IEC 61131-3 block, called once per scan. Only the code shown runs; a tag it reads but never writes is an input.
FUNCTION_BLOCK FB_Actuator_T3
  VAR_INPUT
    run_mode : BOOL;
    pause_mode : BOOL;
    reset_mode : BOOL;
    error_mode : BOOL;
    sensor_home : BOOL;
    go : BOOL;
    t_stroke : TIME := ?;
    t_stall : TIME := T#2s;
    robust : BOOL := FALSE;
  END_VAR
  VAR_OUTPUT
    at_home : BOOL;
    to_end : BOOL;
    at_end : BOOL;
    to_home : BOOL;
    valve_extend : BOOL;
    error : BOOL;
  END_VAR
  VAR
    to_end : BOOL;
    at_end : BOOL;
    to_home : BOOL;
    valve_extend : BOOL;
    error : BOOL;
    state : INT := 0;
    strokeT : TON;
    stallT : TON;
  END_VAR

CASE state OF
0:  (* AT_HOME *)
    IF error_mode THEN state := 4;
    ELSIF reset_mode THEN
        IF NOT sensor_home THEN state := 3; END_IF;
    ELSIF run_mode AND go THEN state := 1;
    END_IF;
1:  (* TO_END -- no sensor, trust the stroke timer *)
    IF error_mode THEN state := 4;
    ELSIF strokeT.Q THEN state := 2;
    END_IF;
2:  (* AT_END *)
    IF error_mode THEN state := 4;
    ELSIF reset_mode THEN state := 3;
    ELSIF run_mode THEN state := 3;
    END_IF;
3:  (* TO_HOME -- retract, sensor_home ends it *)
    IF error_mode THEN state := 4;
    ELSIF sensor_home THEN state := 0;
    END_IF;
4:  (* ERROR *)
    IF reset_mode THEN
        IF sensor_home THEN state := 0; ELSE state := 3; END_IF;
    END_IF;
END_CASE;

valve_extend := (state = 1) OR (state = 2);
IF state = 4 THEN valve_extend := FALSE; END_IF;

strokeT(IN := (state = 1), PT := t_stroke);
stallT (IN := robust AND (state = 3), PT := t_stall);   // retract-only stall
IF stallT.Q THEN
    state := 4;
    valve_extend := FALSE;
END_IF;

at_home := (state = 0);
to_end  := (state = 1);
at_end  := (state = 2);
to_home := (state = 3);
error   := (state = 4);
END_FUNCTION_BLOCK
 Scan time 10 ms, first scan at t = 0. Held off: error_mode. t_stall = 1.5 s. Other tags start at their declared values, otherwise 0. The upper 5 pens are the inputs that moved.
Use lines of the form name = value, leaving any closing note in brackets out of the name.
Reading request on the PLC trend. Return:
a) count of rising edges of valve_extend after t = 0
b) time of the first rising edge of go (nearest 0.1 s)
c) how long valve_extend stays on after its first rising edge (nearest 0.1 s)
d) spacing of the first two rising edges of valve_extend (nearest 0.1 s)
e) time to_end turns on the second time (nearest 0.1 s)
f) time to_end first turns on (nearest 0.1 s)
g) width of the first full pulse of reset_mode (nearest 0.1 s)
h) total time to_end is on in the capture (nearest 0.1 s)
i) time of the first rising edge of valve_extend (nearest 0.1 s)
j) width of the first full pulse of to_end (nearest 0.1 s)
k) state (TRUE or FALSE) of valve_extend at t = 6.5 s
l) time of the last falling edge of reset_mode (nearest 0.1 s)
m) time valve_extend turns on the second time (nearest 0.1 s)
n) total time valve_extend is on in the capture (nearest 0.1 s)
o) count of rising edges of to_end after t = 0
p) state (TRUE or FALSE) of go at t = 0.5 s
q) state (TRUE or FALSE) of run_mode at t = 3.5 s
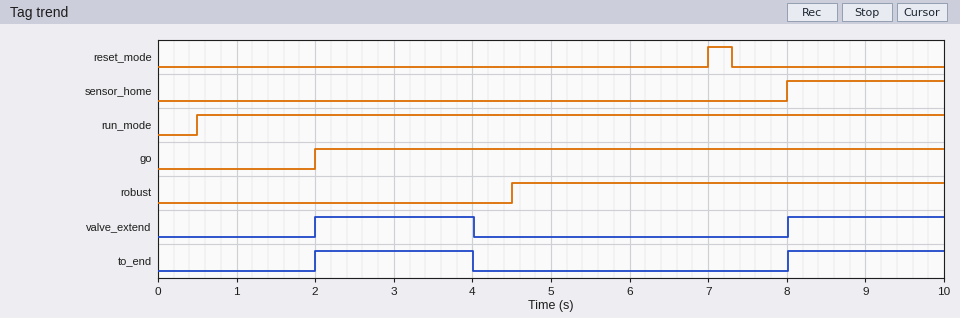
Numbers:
count of rising edges of valve_extend after t = 0 = 2
time of the first rising edge of go = 2.0 s
how long valve_extend stays on after its first rising edge = 2.0 s
spacing of the first two rising edges of valve_extend = 6.0 s
time to_end turns on the second time = 8.0 s
time to_end first turns on = 2.0 s
width of the first full pulse of reset_mode = 0.3 s
total time to_end is on in the capture = 4.0 s
time of the first rising edge of valve_extend = 2.0 s
width of the first full pulse of to_end = 2.0 s
state (TRUE or FALSE) of valve_extend at t = 6.5 s = FALSE
time of the last falling edge of reset_mode = 7.3 s
time valve_extend turns on the second time = 8.0 s
total time valve_extend is on in the capture = 4.0 s
count of rising edges of to_end after t = 0 = 2
state (TRUE or FALSE) of go at t = 0.5 s = FALSE
state (TRUE or FALSE) of run_mode at t = 3.5 s = TRUE
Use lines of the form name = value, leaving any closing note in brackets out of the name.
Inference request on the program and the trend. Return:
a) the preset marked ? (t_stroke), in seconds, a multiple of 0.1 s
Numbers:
the preset marked ? (t_stroke), in seconds, a multiple of 0.1 s = 2.0 s
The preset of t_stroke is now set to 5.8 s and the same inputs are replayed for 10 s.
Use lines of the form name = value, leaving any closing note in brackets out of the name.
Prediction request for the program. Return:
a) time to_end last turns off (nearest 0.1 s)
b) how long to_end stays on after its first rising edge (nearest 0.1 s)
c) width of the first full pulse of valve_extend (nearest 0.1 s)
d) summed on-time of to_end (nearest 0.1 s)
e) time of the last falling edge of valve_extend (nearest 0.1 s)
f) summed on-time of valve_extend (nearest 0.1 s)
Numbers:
time to_end last turns off = 7.8 s
how long to_end stays on after its first rising edge = 5.8 s
width of the first full pulse of valve_extend = 5.8 s
summed on-time of to_end = 7.8 s
time of the last falling edge of valve_extend = 7.8 s
summed on-time of valve_extend = 7.8 s
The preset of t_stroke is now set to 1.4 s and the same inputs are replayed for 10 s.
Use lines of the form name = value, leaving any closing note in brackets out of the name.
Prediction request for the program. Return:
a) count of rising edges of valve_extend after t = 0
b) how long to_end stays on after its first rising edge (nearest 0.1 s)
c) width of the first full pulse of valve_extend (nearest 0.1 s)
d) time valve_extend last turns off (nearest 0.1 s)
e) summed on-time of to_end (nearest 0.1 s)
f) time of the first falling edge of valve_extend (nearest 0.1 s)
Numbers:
count of rising edges of valve_extend after t = 0 = 3
how long to_end stays on after its first rising edge = 1.4 s
width of the first full pulse of valve_extend = 1.4 s
time valve_extend last turns off = 9.4 s
summed on-time of to_end = 3.4 s
time of the first falling edge of valve_extend = 3.4 s
